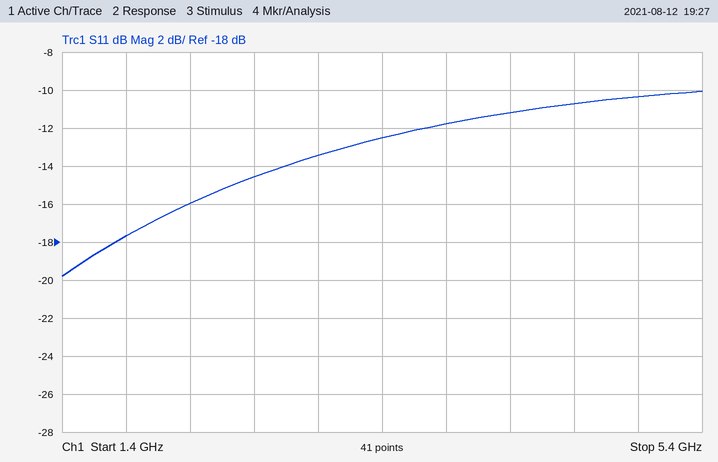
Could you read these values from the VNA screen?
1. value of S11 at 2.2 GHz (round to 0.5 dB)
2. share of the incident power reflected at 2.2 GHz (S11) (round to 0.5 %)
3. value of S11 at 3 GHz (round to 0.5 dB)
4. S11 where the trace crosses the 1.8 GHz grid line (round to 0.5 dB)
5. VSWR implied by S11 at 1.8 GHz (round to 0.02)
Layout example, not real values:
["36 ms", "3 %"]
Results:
["-16.0 dB", "2.5 %", "-13.5 dB", "-17.5 dB", "1.30"]
